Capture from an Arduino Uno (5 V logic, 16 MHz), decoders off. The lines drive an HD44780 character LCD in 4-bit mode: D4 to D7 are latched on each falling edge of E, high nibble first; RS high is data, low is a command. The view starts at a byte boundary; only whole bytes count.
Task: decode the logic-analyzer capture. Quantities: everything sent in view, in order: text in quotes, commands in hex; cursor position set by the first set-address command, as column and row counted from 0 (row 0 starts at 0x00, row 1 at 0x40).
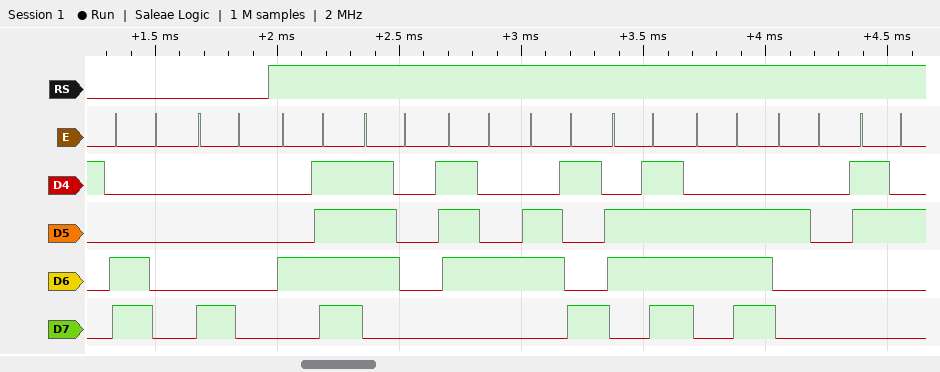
0xC0 0x80 "Option 2"
column 0, row 1
